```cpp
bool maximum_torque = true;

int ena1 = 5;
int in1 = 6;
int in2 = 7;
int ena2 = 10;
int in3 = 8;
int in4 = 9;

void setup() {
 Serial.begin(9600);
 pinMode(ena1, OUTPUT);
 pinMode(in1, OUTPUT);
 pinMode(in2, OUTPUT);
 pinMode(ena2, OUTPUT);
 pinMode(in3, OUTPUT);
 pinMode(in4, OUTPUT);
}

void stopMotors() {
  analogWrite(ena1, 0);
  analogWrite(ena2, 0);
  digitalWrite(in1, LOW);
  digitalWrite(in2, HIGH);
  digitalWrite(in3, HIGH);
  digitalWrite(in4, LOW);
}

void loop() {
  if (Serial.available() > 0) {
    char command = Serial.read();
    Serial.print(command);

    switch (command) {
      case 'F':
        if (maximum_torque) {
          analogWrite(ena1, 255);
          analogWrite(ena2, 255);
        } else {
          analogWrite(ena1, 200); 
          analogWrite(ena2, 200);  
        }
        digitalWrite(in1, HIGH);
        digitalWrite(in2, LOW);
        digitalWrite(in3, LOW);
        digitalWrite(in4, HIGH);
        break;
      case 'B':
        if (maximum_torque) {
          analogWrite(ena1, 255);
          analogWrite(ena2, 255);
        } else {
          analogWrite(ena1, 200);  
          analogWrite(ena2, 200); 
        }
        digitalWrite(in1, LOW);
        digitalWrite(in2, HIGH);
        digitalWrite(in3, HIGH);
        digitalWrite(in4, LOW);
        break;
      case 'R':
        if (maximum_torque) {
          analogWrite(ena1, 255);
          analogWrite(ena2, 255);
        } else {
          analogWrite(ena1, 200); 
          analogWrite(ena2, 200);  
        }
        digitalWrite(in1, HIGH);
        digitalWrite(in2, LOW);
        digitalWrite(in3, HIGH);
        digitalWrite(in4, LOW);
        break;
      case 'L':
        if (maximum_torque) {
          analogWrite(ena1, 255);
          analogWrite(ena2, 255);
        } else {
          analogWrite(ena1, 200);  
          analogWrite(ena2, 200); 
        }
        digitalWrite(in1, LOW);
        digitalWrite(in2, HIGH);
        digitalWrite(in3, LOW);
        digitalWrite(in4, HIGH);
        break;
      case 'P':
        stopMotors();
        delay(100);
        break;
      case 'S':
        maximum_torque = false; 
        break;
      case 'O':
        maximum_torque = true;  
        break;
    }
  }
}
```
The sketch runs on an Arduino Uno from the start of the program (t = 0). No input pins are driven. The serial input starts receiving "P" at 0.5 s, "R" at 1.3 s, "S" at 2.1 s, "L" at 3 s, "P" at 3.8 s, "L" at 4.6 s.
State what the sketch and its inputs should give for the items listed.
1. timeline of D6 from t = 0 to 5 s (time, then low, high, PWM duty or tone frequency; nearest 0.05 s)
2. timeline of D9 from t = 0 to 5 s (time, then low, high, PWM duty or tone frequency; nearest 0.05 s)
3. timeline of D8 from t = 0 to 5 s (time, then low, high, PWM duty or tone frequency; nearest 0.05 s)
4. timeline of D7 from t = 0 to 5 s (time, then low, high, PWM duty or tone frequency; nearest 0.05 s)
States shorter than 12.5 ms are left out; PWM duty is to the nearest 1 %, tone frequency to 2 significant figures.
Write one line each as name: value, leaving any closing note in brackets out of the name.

timeline of D6 from t = 0 to 5 s: 0 s low; 1.3 s high; 3 s low
timeline of D9 from t = 0 to 5 s: 0 s low; 3 s high; 3.8 s low; 4.6 s high
timeline of D8 from t = 0 to 5 s: 0 s low; 0.5 s high; 3 s low; 3.8 s high; 4.6 s low
timeline of D7 from t = 0 to 5 s: 0 s low; 0.5 s high; 1.3 s low; 3 s high
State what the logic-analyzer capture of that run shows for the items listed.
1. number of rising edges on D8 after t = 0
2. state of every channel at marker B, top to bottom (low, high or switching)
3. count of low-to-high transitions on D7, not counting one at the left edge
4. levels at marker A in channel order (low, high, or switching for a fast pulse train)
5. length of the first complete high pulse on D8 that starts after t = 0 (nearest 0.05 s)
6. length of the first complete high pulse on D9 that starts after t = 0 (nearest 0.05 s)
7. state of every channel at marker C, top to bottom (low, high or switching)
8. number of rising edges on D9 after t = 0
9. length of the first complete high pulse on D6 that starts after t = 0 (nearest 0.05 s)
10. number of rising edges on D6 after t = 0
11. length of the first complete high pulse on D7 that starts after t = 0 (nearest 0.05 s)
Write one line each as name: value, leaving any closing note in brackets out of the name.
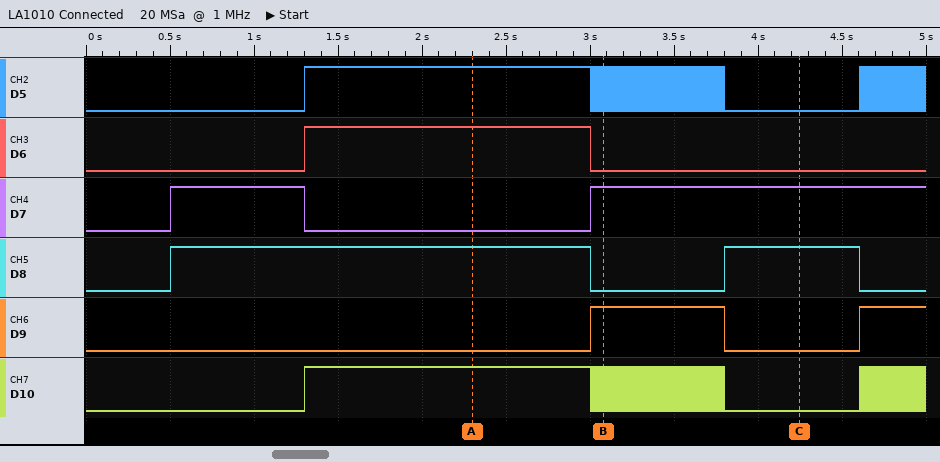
number of rising edges on D8 after t = 0: 2
state of every channel at marker B, top to bottom: D5 switching, D6 low, D7 high, D8 low, D9 high, D10 switching
count of low-to-high transitions on D7, not counting one at the left edge: 2
levels at marker A in channel order: D5 high, D6 high, D7 low, D8 high, D9 low, D10 high
length of the first complete high pulse on D8 that starts after t = 0: 2.50 s
length of the first complete high pulse on D9 that starts after t = 0: 0.80 s
state of every channel at marker C, top to bottom: D5 low, D6 low, D7 high, D8 high, D9 low, D10 low
number of rising edges on D9 after t = 0: 2
length of the first complete high pulse on D6 that starts after t = 0: 1.70 s
number of rising edges on D6 after t = 0: 1
length of the first complete high pulse on D7 that starts after t = 0: 0.80 s
